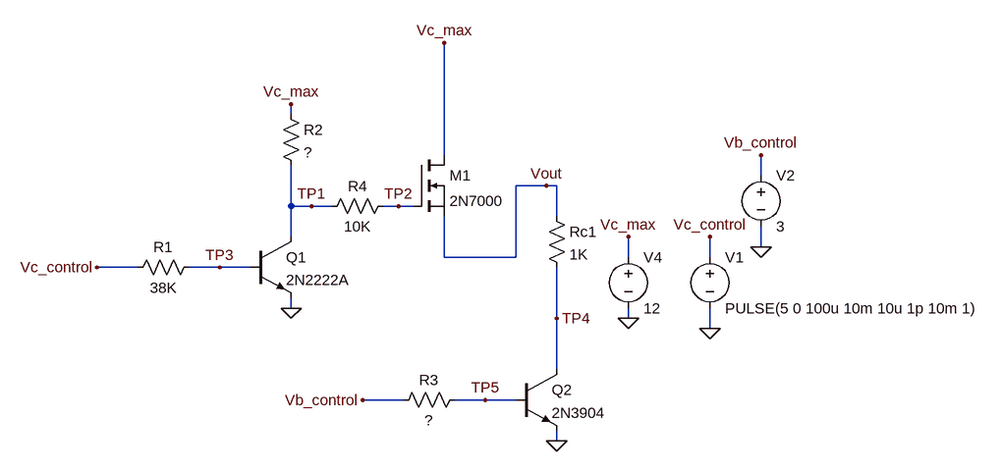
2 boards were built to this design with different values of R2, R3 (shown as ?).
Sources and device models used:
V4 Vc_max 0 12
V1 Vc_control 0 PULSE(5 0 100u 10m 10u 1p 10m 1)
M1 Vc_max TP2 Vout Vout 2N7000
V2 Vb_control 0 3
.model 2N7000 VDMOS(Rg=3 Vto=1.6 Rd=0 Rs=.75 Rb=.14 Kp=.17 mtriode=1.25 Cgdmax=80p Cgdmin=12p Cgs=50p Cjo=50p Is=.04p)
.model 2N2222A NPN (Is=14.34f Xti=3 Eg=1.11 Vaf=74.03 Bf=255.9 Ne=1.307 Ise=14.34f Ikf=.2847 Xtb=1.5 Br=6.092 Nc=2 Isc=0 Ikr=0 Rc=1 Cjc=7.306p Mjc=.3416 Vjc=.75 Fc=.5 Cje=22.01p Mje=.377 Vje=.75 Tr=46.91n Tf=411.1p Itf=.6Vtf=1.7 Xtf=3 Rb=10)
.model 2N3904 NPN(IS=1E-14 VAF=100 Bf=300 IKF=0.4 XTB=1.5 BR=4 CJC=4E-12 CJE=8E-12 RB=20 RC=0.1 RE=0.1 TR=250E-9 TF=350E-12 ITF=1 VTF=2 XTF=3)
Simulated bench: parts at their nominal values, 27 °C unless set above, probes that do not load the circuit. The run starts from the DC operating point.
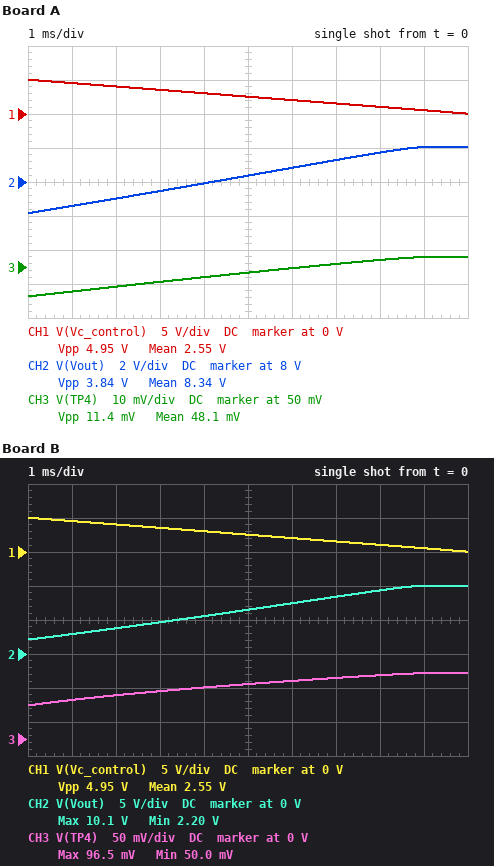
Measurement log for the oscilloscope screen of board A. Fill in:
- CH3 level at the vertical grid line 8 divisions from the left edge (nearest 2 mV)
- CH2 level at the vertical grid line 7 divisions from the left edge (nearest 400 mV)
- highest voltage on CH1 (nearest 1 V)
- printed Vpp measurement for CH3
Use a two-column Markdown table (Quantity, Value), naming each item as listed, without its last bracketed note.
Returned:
| Quantity | Value |
|---|---|
| CH3 level at the vertical grid line 8 divisions from the left edge | 52 mV |
| CH2 level at the vertical grid line 7 divisions from the left edge | 9.2 V |
| highest voltage on CH1 | 5 V |
| printed Vpp measurement for CH3 | 11.4 mV |
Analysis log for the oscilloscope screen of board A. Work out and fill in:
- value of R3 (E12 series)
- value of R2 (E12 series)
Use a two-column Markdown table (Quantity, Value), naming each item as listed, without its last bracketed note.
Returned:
| Quantity | Value |
|---|---|
| value of R3 | 4.7 kΩ |
| value of R2 | 180 Ω |
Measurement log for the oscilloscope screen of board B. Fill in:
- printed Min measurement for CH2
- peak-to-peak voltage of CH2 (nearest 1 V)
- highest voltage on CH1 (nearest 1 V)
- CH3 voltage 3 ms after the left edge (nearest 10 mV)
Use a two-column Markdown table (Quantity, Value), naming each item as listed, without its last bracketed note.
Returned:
| Quantity | Value |
|---|---|
| printed Min measurement for CH2 | 2.20 V |
| peak-to-peak voltage of CH2 | 8 V |
| highest voltage on CH1 | 5 V |
| CH3 voltage 3 ms after the left edge | 70 mV |
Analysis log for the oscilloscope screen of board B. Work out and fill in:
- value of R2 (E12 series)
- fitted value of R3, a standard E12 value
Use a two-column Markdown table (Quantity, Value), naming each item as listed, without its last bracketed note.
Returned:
| Quantity | Value |
|---|---|
| value of R2 | 390 Ω |
| fitted value of R3, a standard E12 value | 22 kΩ |
